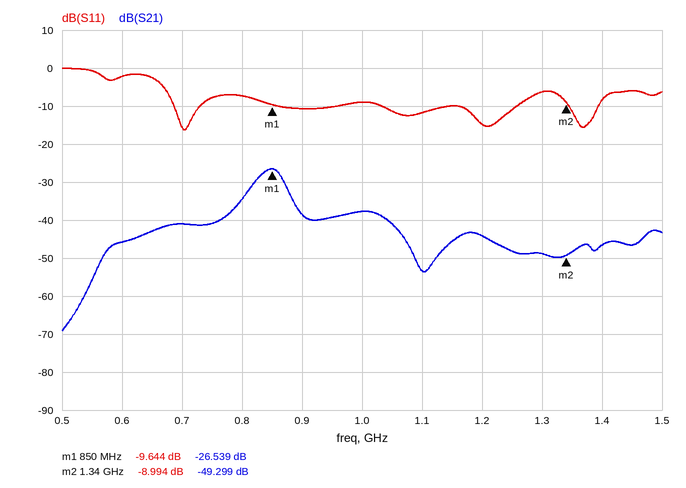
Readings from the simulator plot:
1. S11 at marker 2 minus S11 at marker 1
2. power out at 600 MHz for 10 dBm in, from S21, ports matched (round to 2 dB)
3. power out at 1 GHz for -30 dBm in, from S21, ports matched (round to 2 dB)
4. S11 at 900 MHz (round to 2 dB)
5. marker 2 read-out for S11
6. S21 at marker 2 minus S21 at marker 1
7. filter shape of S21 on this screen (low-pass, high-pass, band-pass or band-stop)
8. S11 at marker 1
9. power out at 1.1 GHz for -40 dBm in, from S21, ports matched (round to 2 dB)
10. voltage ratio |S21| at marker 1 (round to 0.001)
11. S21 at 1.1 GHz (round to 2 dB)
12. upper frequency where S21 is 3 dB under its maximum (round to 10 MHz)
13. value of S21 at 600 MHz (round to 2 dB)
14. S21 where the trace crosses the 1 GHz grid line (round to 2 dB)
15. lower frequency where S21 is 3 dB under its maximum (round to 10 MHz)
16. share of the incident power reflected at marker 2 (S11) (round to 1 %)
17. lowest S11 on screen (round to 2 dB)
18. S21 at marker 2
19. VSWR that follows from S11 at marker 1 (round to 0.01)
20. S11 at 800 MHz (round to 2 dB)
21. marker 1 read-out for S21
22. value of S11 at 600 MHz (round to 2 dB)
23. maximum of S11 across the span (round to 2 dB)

0.650 dB
-36 dBm
-68 dBm
-10 dB
-8.994 dB
-22.760 dB
band-pass
-9.644 dB
-94 dBm
0.047
-54 dB
870 MHz
-46 dB
-38 dB
820 MHz
13 %
-16 dB
-49.299 dB
1.98
-8 dB
-26.539 dB
-2 dB
0 dB
